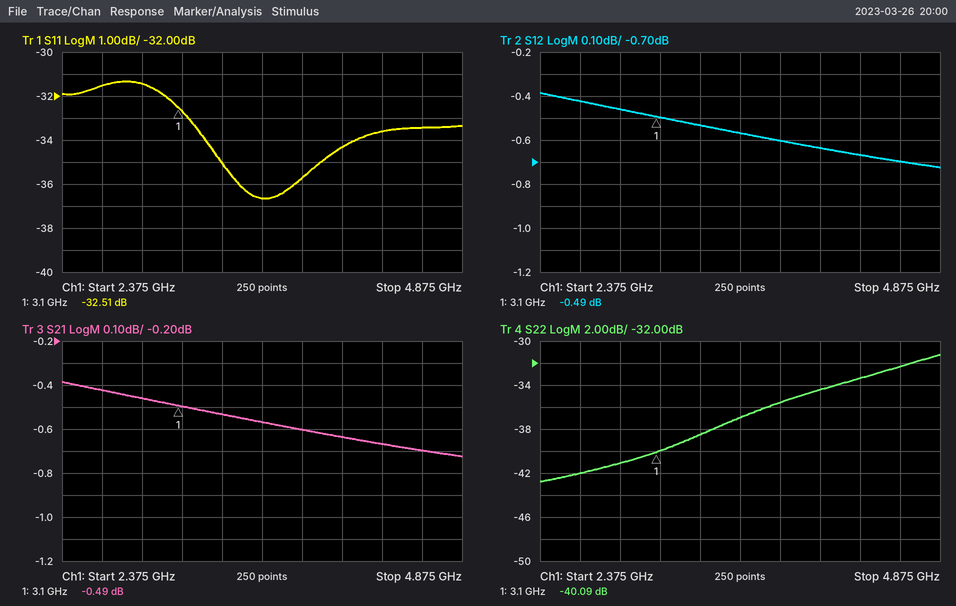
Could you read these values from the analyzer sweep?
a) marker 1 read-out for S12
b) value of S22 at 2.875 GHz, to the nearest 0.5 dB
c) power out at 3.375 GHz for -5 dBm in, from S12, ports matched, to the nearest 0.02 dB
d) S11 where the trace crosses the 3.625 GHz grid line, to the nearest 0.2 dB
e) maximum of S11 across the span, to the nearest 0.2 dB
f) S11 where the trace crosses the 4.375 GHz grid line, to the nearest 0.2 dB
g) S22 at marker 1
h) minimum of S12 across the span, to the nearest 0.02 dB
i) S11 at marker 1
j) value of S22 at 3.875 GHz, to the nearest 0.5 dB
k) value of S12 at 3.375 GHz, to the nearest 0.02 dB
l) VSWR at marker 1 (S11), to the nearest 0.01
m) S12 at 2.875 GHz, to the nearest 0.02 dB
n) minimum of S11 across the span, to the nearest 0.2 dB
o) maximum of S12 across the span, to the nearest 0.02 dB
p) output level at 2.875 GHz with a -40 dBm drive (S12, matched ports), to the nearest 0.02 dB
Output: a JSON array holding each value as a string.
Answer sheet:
["-0.49 dB", "-41.0 dB", "-5.54 dBm", "-36.6 dB", "-31.4 dB", "-33.6 dB", "-40.09 dB", "-0.72 dB", "-32.51 dB", "-35.5 dB", "-0.54 dB", "1.05", "-0.46 dB", "-36.6 dB", "-0.38 dB", "-40.46 dBm"]
